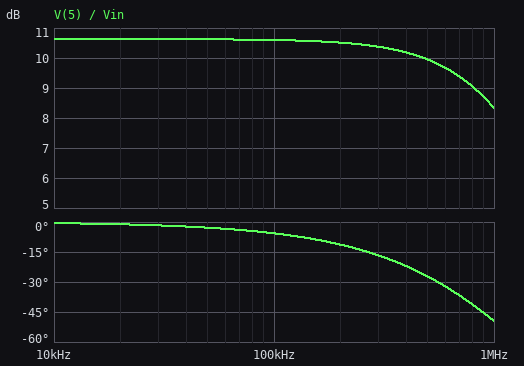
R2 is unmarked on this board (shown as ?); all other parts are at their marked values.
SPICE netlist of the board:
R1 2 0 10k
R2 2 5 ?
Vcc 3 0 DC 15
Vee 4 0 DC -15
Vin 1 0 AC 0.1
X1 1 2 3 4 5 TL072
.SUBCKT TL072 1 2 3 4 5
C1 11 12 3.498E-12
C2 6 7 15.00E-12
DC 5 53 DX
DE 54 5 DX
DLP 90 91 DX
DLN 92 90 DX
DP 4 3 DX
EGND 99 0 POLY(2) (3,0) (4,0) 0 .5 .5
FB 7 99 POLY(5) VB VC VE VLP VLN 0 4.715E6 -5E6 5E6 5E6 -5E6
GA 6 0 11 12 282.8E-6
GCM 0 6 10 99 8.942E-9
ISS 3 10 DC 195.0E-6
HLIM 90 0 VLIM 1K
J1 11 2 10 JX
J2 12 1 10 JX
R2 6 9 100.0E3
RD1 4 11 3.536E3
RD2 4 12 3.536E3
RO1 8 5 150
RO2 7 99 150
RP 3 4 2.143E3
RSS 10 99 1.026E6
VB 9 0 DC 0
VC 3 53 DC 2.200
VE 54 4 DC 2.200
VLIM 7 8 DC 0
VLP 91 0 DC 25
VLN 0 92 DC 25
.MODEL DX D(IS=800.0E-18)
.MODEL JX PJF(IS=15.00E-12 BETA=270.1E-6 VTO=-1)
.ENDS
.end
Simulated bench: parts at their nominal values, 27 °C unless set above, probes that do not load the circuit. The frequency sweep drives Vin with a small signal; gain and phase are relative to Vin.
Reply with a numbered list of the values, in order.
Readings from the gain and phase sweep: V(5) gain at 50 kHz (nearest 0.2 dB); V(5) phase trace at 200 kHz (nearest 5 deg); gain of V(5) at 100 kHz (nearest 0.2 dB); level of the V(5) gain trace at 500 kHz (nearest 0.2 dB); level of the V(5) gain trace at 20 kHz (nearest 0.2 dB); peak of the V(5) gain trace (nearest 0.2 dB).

1. 10.6 dB
2. -10 deg
3. 10.6 dB
4. 10.0 dB
5. 10.6 dB
6. 10.6 dB
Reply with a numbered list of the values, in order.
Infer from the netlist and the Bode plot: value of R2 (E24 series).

1. 24 kΩ
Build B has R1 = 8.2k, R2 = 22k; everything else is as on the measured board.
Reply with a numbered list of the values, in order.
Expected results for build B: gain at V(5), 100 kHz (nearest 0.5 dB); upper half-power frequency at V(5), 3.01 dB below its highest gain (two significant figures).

1. 11.5 dB
2. 1.1 MHz
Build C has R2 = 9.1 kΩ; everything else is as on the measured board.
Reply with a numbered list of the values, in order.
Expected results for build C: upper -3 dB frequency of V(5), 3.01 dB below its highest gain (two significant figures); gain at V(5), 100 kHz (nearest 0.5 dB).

1. 2.4 MHz
2. 5.5 dB
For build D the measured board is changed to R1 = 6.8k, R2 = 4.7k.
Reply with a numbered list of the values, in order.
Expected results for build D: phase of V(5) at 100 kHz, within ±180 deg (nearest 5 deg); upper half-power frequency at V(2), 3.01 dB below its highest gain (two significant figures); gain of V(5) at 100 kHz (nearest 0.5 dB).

1. -5 deg
2. 2.7 MHz
3. 4.5 dB
